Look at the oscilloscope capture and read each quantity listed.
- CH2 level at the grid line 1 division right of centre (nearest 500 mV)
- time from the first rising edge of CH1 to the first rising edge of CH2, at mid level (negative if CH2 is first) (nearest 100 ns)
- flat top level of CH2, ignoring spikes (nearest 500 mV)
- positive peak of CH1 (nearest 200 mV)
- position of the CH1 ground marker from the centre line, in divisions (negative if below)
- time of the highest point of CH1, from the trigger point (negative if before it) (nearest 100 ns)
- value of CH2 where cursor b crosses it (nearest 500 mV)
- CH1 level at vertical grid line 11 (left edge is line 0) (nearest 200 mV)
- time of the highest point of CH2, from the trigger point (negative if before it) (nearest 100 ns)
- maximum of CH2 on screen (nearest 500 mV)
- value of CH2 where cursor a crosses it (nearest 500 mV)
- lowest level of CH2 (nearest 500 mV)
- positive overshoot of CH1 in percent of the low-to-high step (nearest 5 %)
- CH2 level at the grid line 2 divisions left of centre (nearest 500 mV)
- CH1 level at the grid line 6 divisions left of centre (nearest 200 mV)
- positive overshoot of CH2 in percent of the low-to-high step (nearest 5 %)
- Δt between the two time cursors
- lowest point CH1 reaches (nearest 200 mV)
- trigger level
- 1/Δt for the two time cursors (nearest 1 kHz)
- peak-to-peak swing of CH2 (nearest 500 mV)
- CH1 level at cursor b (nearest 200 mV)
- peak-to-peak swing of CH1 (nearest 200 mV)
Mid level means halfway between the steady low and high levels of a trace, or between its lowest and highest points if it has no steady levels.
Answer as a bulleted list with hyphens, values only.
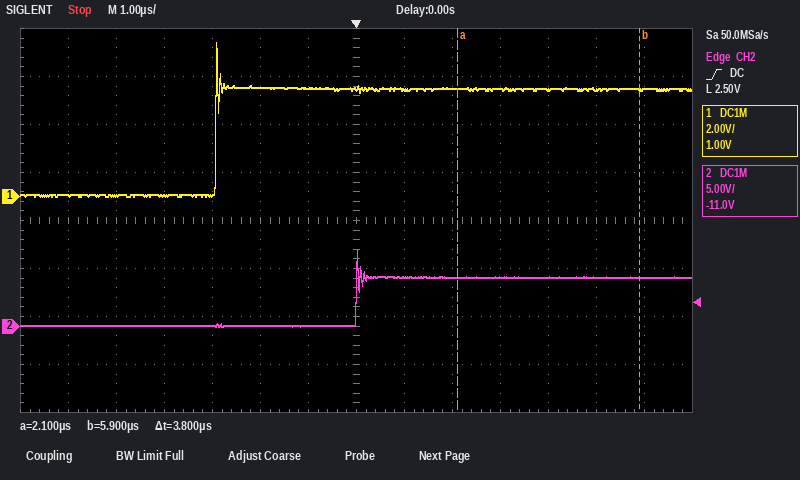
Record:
- 5.0 V
- +2.9 µs
- 5.0 V
- 6.4 V
- +0.5 div
- -2.9 µs
- 5.0 V
- 4.4 V
- 0.0 µs
- 8.0 V
- 5.0 V
- 0.0 V
- 45 %
- 0.0 V
- 0.0 V
- 60 %
- 3.8 µs
- 0.0 V
- 2.50 V
- 263 kHz
- 8.0 V
- 4.4 V
- 6.4 V
